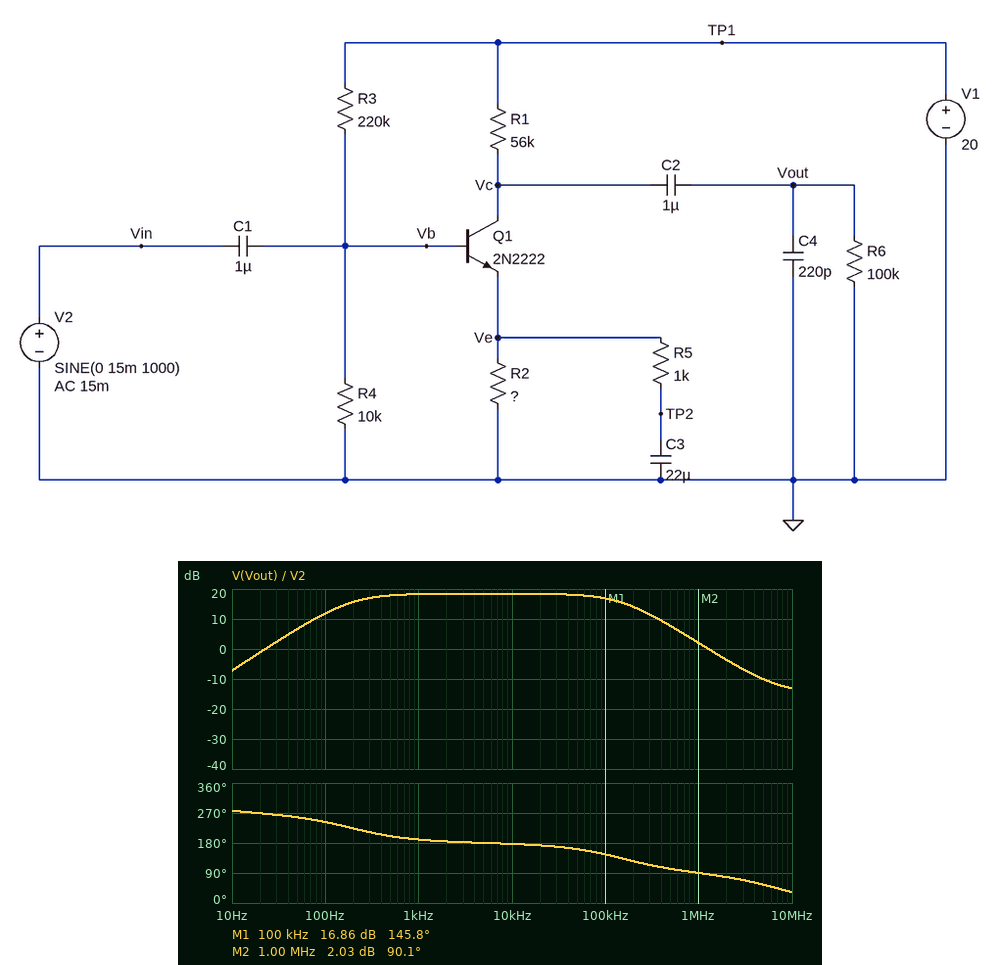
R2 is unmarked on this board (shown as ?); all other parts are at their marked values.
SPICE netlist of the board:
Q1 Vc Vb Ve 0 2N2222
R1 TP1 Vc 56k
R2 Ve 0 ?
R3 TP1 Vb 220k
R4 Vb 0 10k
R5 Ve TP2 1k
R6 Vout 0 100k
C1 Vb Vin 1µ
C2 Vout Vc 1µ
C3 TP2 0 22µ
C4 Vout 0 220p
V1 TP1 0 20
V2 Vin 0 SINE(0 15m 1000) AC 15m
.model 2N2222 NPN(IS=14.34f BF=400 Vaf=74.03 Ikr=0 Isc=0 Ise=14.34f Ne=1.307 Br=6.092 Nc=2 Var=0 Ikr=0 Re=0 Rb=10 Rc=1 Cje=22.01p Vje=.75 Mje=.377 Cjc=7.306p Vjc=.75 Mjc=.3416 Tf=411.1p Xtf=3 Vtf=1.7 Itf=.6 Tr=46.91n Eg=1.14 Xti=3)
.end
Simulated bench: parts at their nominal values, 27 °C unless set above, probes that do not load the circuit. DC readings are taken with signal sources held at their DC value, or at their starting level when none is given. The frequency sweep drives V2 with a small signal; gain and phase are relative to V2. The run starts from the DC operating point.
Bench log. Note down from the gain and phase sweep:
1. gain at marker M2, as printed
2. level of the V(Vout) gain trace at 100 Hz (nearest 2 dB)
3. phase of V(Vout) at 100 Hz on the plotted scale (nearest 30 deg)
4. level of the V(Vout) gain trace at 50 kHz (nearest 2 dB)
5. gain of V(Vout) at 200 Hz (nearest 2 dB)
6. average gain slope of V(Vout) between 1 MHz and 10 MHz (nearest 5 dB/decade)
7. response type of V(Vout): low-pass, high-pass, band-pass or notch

2.03 dB
12 dB
240 deg
18 dB
16 dB
-15 dB/decade
band-pass
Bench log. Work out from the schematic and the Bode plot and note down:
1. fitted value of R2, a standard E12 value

560 Ω
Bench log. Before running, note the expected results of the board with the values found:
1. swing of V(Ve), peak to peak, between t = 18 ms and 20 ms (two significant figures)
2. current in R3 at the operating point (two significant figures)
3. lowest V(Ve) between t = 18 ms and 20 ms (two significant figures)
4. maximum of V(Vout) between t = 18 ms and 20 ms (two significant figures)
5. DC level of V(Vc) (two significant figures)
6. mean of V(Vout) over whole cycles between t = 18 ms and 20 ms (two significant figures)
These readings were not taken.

20 mV
87 µA
180 mV
1.4 V
280 mV
430 mV
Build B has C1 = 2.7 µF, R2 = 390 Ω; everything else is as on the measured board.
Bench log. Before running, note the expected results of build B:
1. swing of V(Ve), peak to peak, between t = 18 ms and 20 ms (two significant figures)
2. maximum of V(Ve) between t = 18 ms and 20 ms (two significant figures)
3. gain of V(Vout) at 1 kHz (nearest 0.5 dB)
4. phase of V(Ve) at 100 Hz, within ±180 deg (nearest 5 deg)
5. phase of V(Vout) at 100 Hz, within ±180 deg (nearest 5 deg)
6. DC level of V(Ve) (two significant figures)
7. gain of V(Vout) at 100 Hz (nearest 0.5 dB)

16 mV
150 mV
9.5 dB
40 deg
-140 deg
140 mV
7.0 dB
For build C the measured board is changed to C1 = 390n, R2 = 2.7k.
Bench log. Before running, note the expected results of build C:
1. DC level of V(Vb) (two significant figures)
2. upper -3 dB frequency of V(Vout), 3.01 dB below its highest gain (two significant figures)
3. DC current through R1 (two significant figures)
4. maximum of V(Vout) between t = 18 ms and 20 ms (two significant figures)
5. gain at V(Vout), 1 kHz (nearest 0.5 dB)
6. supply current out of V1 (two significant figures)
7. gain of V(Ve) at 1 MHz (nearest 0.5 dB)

860 mV
20 kHz
100 µA
530 mV
31.0 dB
190 µA
-2.5 dB
